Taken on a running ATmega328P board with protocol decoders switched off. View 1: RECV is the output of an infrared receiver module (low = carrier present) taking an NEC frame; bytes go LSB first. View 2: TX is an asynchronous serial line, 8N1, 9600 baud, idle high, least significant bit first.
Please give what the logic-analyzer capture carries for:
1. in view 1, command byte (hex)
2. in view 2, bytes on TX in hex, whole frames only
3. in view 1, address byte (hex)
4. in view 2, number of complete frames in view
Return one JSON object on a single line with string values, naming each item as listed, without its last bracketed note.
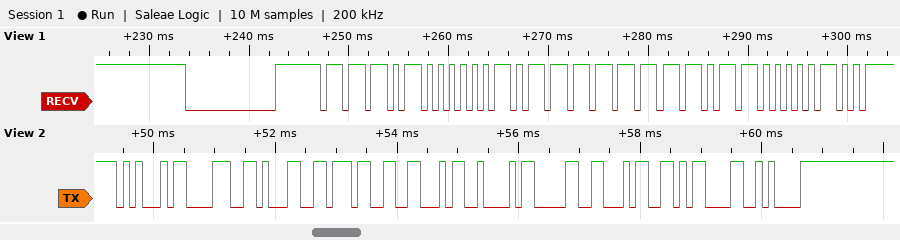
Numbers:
{"in view 1, command byte": "0xDF", "in view 2, bytes on TX in hex, whole frames only": "0x45 0x38 0x31 0x37 0x46 0x42 0x30 0x34 0x0D 0x0A", "in view 1, address byte": "0x17", "in view 2, number of complete frames in view": "10"}
